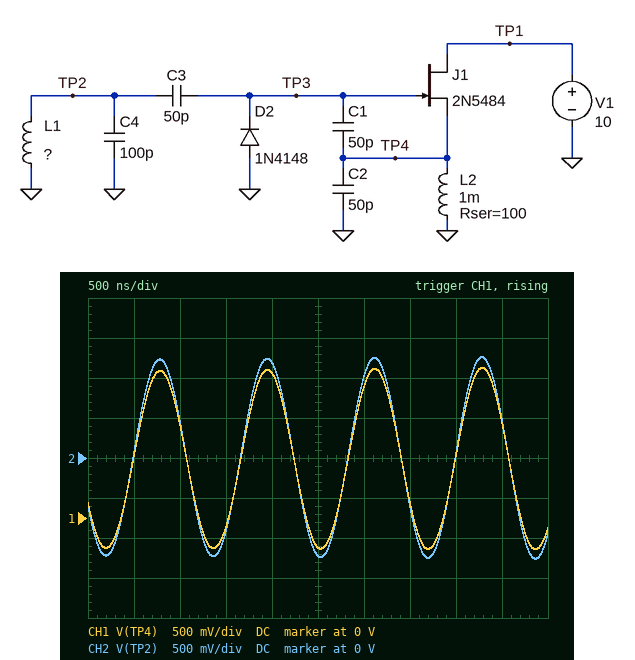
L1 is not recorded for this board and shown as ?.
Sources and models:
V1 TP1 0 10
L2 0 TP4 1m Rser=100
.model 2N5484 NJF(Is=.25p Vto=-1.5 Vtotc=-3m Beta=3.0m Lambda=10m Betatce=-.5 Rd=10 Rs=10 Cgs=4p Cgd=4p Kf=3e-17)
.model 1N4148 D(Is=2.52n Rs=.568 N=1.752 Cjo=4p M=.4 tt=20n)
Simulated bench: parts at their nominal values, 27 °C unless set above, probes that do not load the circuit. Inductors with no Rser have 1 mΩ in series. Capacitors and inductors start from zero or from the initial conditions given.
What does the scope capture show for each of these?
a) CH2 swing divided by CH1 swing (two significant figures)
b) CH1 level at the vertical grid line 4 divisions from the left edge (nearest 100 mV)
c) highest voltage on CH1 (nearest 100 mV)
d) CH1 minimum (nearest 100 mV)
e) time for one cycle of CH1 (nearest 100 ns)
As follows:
1.1
1.8 V
1.9 V
-400 mV
1.2 µs
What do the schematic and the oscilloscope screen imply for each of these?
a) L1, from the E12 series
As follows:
330 µH
